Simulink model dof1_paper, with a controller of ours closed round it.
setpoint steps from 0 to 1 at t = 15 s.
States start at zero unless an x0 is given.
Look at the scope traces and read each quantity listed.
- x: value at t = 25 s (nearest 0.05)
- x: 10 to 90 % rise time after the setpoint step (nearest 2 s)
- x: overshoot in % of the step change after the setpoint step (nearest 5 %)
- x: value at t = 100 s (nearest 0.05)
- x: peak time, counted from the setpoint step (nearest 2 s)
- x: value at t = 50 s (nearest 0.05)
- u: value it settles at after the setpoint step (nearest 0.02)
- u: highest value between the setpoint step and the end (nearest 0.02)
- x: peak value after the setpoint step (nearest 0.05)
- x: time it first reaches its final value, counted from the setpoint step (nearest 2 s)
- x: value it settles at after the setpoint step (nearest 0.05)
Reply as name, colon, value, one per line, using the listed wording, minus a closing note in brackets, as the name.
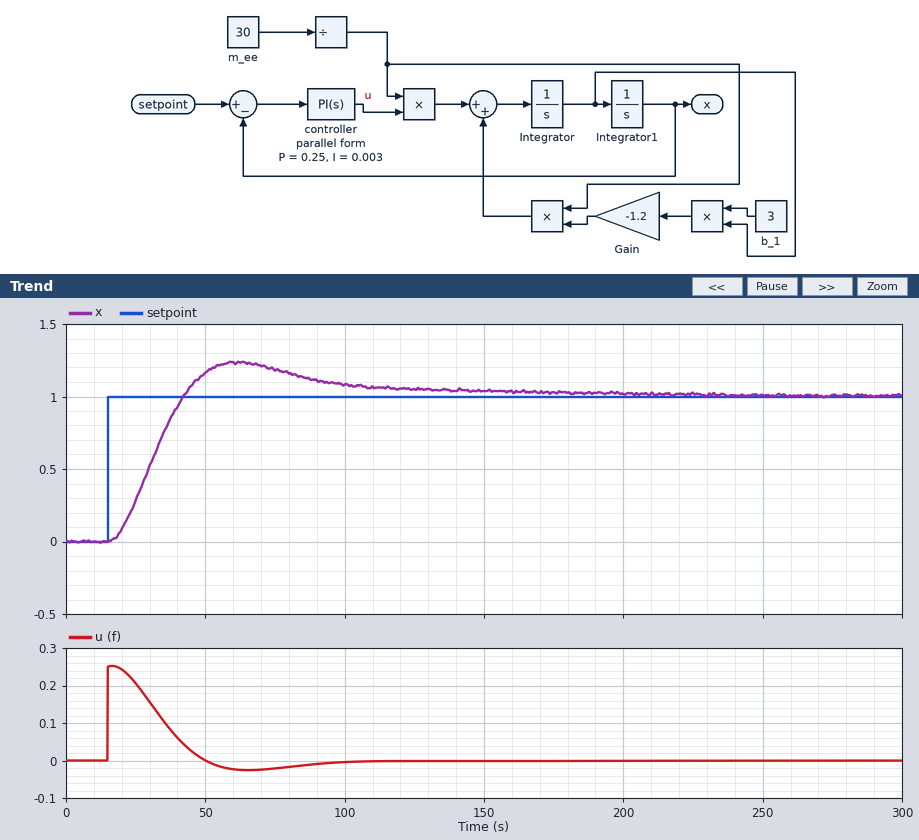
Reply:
x: value at t = 25 s: 0.30
x: 10 to 90 % rise time after the setpoint step: 18 s
x: overshoot in % of the step change after the setpoint step: 25 %
x: value at t = 100 s: 1.10
x: peak time, counted from the setpoint step: 46 s
x: value at t = 50 s: 1.15
u: value it settles at after the setpoint step: 0.00
u: highest value between the setpoint step and the end: 0.26
x: peak value after the setpoint step: 1.25
x: time it first reaches its final value, counted from the setpoint step: 28 s
x: value it settles at after the setpoint step: 1.00
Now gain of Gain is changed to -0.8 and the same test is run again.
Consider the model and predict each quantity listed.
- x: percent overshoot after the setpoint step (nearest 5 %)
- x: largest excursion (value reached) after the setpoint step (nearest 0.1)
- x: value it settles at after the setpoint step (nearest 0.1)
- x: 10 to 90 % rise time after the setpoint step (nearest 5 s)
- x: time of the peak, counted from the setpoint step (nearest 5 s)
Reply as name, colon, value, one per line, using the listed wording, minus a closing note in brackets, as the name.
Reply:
x: percent overshoot after the setpoint step: 40 %
x: largest excursion (value reached) after the setpoint step: 1.4
x: value it settles at after the setpoint step: 1.0
x: 10 to 90 % rise time after the setpoint step: 15 s
x: time of the peak, counted from the setpoint step: 40 s
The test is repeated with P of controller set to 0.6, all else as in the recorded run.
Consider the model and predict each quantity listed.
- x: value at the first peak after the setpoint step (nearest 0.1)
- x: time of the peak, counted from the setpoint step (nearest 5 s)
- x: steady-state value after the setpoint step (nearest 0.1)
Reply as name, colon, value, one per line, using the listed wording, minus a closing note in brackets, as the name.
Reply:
x: value at the first peak after the setpoint step: 1.3
x: time of the peak, counted from the setpoint step: 25 s
x: steady-state value after the setpoint step: 1.0
